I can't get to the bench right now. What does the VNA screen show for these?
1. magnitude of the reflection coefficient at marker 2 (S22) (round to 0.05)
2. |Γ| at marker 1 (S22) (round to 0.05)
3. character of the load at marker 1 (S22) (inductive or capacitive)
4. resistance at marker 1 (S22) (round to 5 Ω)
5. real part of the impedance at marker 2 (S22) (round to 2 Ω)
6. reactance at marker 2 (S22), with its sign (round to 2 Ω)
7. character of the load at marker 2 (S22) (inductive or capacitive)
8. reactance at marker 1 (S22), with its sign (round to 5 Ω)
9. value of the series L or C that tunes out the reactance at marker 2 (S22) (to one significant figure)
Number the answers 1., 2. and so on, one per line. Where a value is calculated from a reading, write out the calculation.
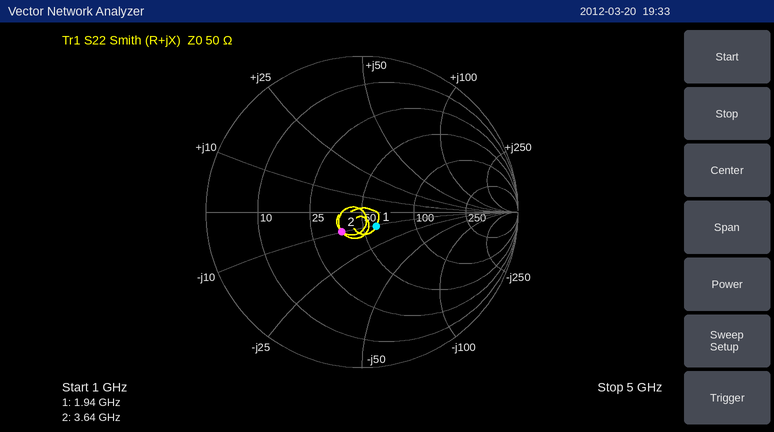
1. 0.20
2. 0.15
3. capacitive
4. 60 Ω
5. 38 Ω
6. -10 Ω
7. capacitive
8. -10 Ω
9. L = 10 Ω/(2π × 3.64 GHz) ≈ 437 pH, so 400 pH to one significant figure
